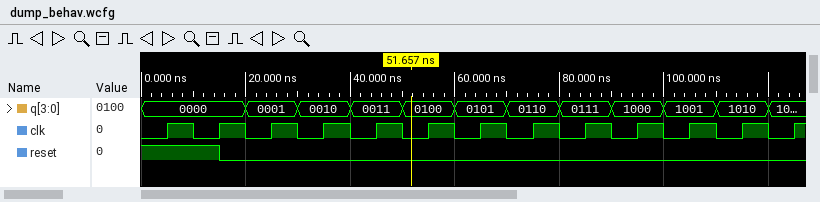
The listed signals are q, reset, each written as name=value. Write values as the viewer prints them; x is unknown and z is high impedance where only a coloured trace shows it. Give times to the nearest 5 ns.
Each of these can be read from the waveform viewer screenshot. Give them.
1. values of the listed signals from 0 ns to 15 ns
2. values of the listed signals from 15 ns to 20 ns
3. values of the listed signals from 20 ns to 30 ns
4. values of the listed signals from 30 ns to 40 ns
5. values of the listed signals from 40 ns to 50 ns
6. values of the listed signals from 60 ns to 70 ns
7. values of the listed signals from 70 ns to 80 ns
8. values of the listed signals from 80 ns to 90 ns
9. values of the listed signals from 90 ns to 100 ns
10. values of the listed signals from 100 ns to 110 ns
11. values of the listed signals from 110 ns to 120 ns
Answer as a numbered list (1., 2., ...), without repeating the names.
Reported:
1. q=0000, reset=1
2. q=0000, reset=0
3. q=0001, reset=0
4. q=0010, reset=0
5. q=0011, reset=0
6. q=0101, reset=0
7. q=0110, reset=0
8. q=0111, reset=0
9. q=1000, reset=0
10. q=1001, reset=0
11. q=1010, reset=0
